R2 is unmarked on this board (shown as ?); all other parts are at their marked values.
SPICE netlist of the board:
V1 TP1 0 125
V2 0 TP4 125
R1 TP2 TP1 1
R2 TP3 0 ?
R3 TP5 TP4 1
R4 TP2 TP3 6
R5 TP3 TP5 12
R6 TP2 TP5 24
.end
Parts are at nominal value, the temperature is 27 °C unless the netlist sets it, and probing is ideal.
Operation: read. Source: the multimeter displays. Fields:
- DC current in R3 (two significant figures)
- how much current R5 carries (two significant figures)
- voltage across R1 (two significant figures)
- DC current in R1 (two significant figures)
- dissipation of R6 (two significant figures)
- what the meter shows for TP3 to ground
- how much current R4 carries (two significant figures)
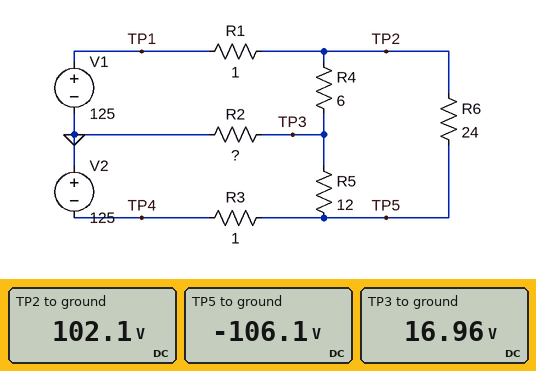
19 A
10 A
23 V
23 A
1.8 kW
16.96 V
14 A
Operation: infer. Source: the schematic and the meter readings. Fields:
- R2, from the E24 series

4.3 Ω
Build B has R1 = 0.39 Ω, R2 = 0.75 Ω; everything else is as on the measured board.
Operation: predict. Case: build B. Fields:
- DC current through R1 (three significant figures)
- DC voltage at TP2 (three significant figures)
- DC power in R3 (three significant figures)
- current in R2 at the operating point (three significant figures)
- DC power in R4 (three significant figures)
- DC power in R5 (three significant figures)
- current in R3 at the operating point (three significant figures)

27.2 A
114 V
346 W
8.59 A
1.94 kW
1.06 kW
18.6 A
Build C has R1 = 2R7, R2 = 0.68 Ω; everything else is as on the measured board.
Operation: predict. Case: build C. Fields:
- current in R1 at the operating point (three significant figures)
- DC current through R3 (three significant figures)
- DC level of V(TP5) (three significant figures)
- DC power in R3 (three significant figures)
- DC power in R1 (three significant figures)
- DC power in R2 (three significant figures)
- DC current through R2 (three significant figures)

19.4 A
16.7 A
-108 V
279 W
1.01 kW
4.76 W
2.65 A
